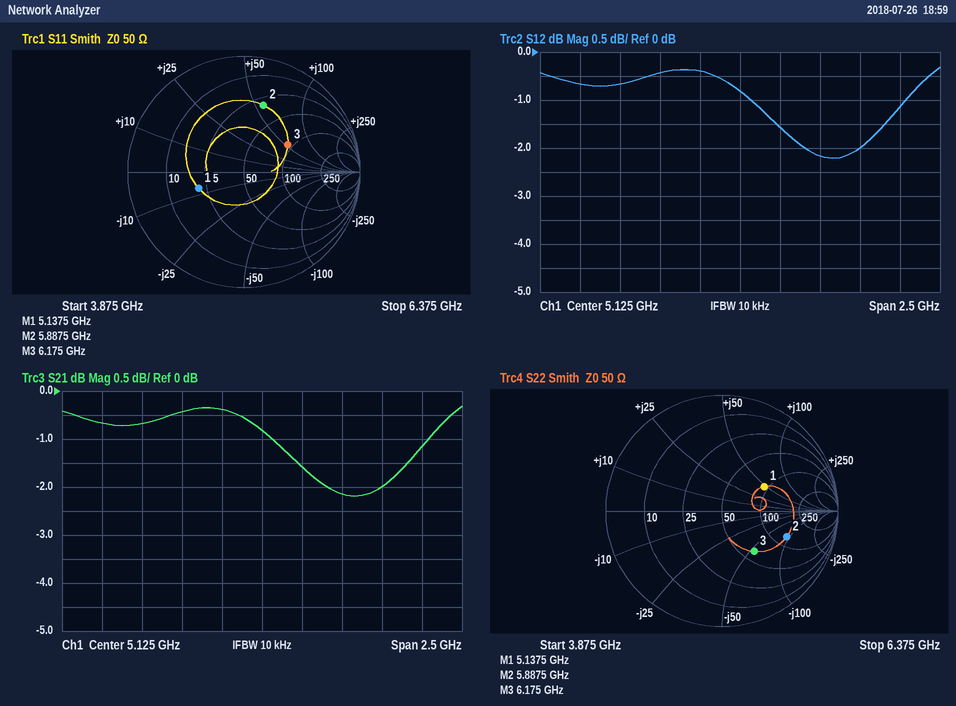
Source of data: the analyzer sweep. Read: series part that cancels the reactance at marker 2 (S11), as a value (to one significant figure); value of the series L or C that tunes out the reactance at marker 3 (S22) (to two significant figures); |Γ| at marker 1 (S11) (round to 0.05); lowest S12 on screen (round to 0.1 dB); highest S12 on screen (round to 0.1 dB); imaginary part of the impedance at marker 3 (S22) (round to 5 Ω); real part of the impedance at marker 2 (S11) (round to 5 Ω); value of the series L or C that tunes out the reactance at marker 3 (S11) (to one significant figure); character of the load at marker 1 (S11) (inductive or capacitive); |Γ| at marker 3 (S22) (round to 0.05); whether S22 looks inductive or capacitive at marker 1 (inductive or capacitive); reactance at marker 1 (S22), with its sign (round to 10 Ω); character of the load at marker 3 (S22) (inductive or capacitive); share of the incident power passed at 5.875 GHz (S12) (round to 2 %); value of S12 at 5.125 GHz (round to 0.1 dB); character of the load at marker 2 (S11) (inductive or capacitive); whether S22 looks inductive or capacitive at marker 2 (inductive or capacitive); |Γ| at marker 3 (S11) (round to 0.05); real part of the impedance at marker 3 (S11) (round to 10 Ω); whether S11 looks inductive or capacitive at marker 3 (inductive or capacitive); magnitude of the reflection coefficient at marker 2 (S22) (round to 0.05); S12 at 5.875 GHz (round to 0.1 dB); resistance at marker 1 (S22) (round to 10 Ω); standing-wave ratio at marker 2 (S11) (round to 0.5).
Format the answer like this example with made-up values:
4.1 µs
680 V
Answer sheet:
500 fF
1.4 nH
0.40
-2.2 dB
-0.3 dB
-55 Ω
30 Ω
500 fF
capacitive
0.45
inductive
+50 Ω
capacitive
64 %
-0.8 dB
inductive
capacitive
0.45
90 Ω
inductive
0.60
-2.0 dB
90 Ω
4.0
